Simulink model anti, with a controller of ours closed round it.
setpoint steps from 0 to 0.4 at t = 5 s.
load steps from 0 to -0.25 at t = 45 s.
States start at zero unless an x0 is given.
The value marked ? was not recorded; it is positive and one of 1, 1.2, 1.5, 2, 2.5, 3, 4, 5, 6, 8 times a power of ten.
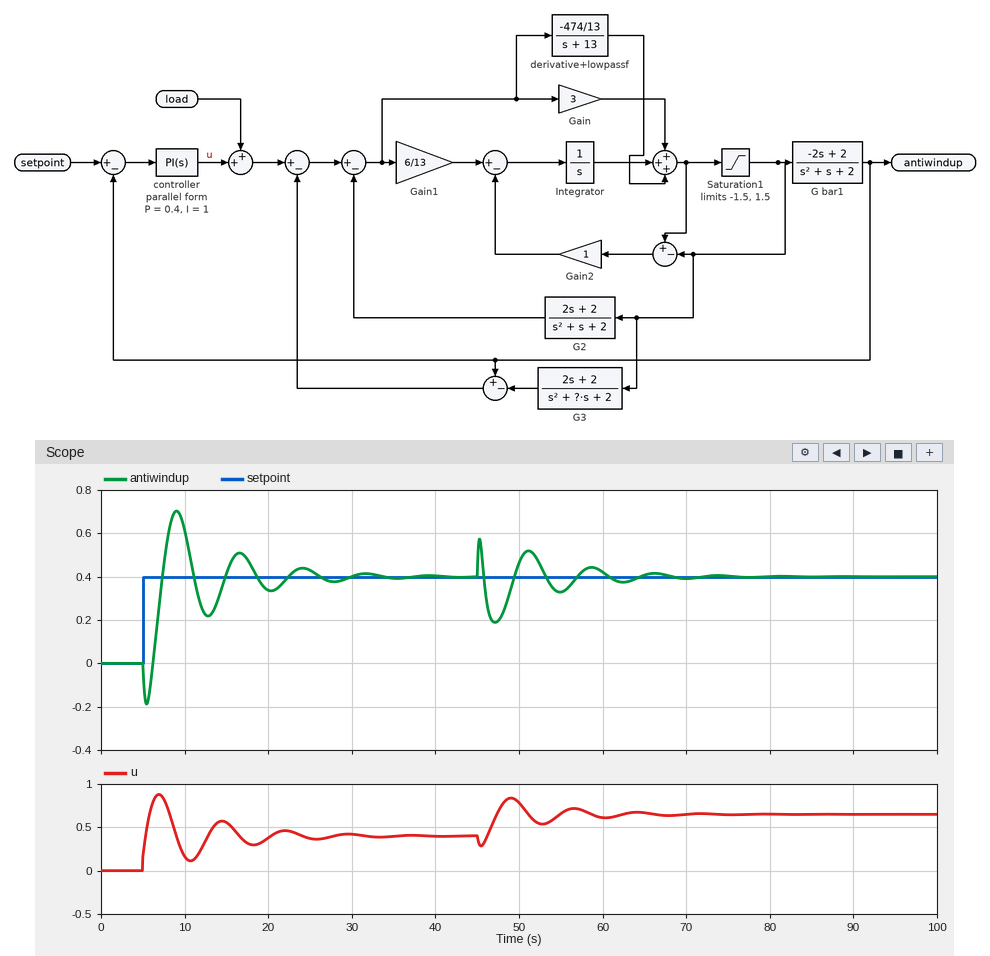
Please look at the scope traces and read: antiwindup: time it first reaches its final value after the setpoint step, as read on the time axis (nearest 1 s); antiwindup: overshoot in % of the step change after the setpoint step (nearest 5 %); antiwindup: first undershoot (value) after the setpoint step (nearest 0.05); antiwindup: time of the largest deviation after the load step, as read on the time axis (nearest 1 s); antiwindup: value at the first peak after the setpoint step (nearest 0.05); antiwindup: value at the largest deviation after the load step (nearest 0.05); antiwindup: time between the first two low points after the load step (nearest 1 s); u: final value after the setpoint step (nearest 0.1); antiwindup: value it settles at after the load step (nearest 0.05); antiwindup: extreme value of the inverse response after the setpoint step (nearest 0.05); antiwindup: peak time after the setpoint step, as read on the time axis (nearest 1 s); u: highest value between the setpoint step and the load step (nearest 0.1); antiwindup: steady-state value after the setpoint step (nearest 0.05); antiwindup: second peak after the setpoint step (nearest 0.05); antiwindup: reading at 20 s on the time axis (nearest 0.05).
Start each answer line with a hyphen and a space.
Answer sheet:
- 7 s
- 75 %
- 0.20
- 47 s
- 0.70
- 0.20
- 8 s
- 0.4
- 0.40
- -0.20
- 9 s
- 0.9
- 0.40
- 0.50
- 0.35
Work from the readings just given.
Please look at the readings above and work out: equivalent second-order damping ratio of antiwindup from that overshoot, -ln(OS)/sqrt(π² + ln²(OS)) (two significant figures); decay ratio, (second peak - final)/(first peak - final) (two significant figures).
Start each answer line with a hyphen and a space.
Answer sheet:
- 0.091
- 0.33
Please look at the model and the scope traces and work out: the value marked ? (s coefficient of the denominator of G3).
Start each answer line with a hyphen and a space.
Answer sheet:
- 2
